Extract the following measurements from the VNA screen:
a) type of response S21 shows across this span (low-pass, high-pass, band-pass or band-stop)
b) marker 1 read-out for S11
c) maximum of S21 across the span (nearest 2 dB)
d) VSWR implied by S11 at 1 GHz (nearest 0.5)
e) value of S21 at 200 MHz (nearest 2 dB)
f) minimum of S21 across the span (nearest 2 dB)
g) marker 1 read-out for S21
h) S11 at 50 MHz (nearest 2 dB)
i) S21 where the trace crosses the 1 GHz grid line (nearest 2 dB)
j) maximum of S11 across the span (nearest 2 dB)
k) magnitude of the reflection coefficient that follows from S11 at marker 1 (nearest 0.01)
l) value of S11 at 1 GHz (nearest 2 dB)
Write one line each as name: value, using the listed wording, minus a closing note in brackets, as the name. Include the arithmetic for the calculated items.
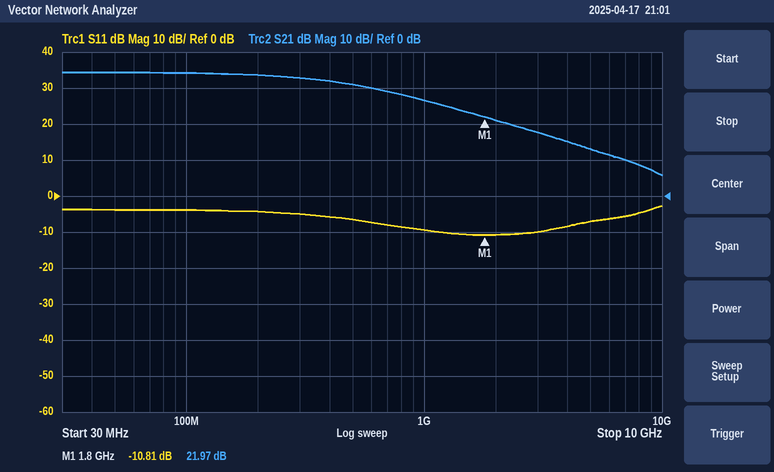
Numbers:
type of response S21 shows across this span: low-pass
marker 1 read-out for S11: -10.81 dB
maximum of S21 across the span: 34 dB
VSWR implied by S11 at 1 GHz: |Γ| = 10^(-10/20) = 0.3162; VSWR = (1 + 0.3162)/(1 − 0.3162) ≈ 1.92, so 2.0 to the nearest 0.5
value of S21 at 200 MHz: 34 dB
minimum of S21 across the span: 6 dB
marker 1 read-out for S21: 21.97 dB
S11 at 50 MHz: -4 dB
S21 where the trace crosses the 1 GHz grid line: 26 dB
maximum of S11 across the span: -2 dB
magnitude of the reflection coefficient that follows from S11 at marker 1: 10^(-10.81/20) ≈ 0.29
value of S11 at 1 GHz: -10 dB
